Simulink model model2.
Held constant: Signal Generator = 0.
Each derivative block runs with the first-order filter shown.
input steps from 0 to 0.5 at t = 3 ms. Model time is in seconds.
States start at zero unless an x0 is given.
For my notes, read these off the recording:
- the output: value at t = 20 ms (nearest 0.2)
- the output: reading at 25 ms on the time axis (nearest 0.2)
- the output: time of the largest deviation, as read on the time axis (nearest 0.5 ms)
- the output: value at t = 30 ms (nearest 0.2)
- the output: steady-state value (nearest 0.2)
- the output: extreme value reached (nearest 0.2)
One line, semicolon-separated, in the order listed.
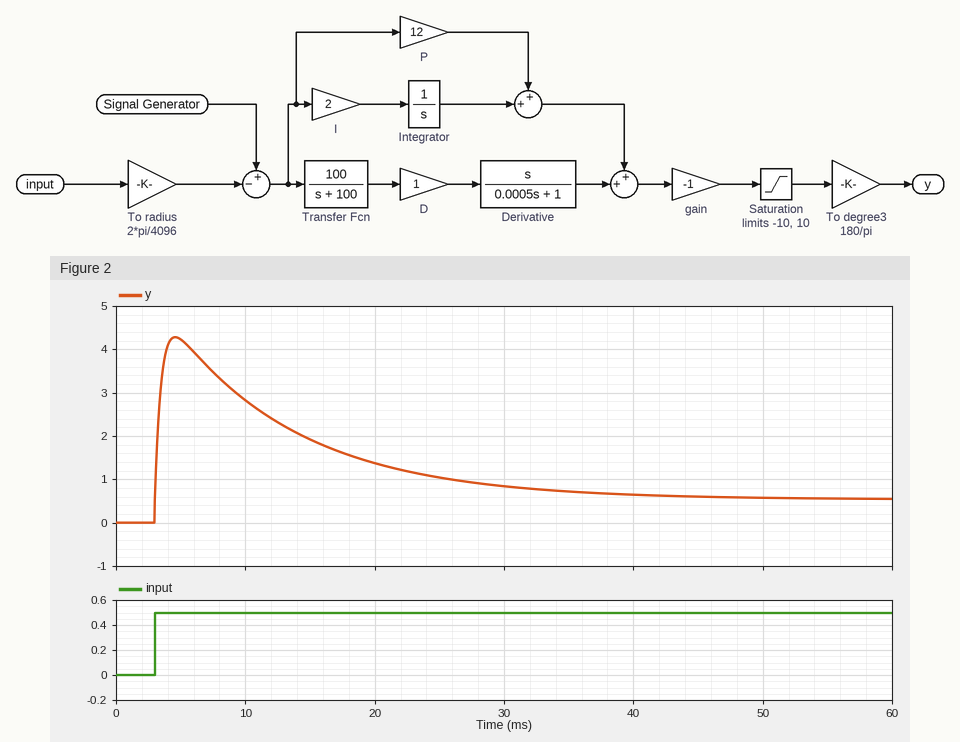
1.4; 1.0; 4.5 ms; 0.8; 0.6; 4.2
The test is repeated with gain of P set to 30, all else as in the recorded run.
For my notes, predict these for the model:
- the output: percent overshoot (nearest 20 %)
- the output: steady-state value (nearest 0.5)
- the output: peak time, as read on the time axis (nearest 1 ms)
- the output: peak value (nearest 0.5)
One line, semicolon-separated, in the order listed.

280 %; 1.5; 5 ms; 5.0
